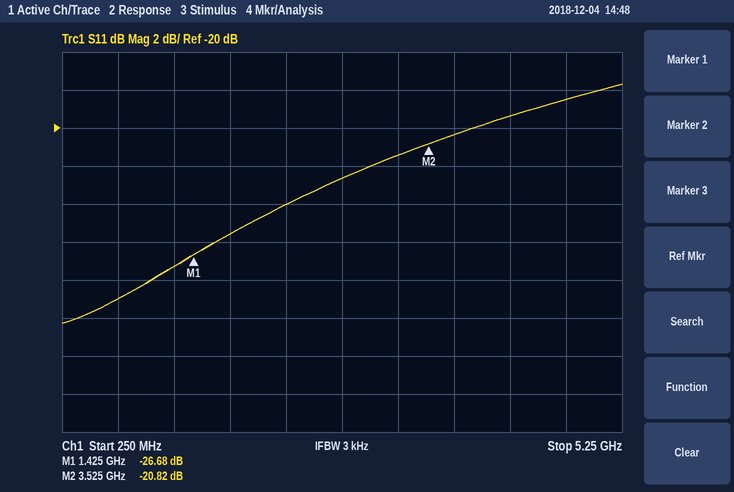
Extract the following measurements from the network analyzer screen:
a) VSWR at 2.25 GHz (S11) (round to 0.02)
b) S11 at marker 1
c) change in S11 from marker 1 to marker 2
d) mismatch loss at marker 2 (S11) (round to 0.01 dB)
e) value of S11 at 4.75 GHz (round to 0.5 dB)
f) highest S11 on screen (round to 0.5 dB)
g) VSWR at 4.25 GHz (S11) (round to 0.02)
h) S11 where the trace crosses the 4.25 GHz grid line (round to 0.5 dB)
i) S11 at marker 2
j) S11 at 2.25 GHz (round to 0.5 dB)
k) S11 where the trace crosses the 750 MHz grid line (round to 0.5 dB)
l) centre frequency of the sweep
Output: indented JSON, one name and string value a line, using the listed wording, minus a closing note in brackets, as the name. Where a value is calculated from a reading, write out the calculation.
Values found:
{
  "VSWR at 2.25 GHz (S11)": "|Γ| = 10^(-24/20) = 0.0631; VSWR = (1 + 0.0631)/(1 − 0.0631) ≈ 1.13, so 1.14 to the nearest 0.02",
  "S11 at marker 1": "-26.68 dB",
  "change in S11 from marker 1 to marker 2": "-20.82 − (-26.68) = 5.86 dB",
  "mismatch loss at marker 2 (S11)": "−10 log10(1 − 10^(-20.82/10)) ≈ 0.04 dB",
  "value of S11 at 4.75 GHz": "-18.5 dB",
  "highest S11 on screen": "-17.5 dB",
  "VSWR at 4.25 GHz (S11)": "|Γ| = 10^(-19.5/20) = 0.1059; VSWR = (1 + 0.1059)/(1 − 0.1059) ≈ 1.24",
  "S11 where the trace crosses the 4.25 GHz grid line": "-19.5 dB",
  "S11 at marker 2": "-20.82 dB",
  "S11 at 2.25 GHz": "-24.0 dB",
  "S11 where the trace crosses the 750 MHz grid line": "-29.0 dB",
  "centre frequency of the sweep": "2.75 GHz"
}
